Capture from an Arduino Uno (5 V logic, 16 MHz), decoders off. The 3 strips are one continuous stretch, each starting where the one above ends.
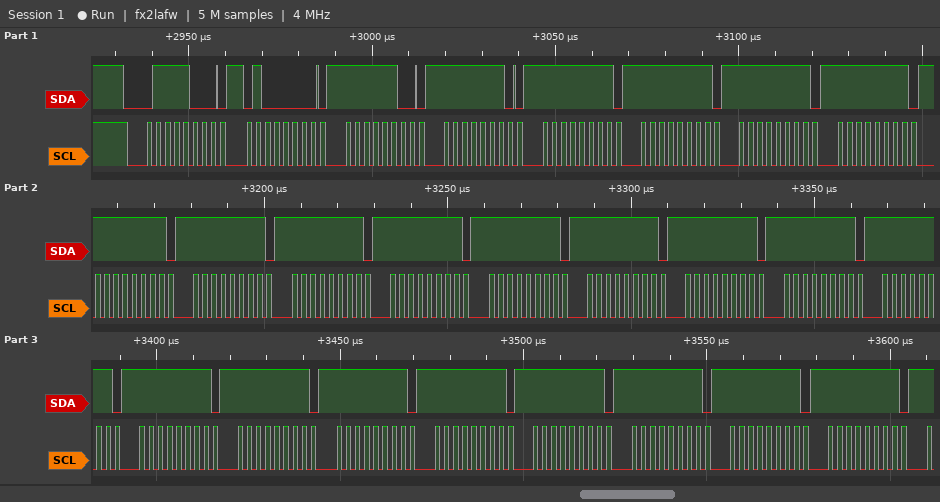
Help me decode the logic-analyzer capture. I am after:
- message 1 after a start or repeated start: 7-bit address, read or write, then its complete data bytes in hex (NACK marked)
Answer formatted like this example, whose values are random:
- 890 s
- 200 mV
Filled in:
- 0x3C write: 40 FC FE FF FF FF FF FF FF FF FF FF FF FF FF FF FF FF FF FF FF FF FF FF
